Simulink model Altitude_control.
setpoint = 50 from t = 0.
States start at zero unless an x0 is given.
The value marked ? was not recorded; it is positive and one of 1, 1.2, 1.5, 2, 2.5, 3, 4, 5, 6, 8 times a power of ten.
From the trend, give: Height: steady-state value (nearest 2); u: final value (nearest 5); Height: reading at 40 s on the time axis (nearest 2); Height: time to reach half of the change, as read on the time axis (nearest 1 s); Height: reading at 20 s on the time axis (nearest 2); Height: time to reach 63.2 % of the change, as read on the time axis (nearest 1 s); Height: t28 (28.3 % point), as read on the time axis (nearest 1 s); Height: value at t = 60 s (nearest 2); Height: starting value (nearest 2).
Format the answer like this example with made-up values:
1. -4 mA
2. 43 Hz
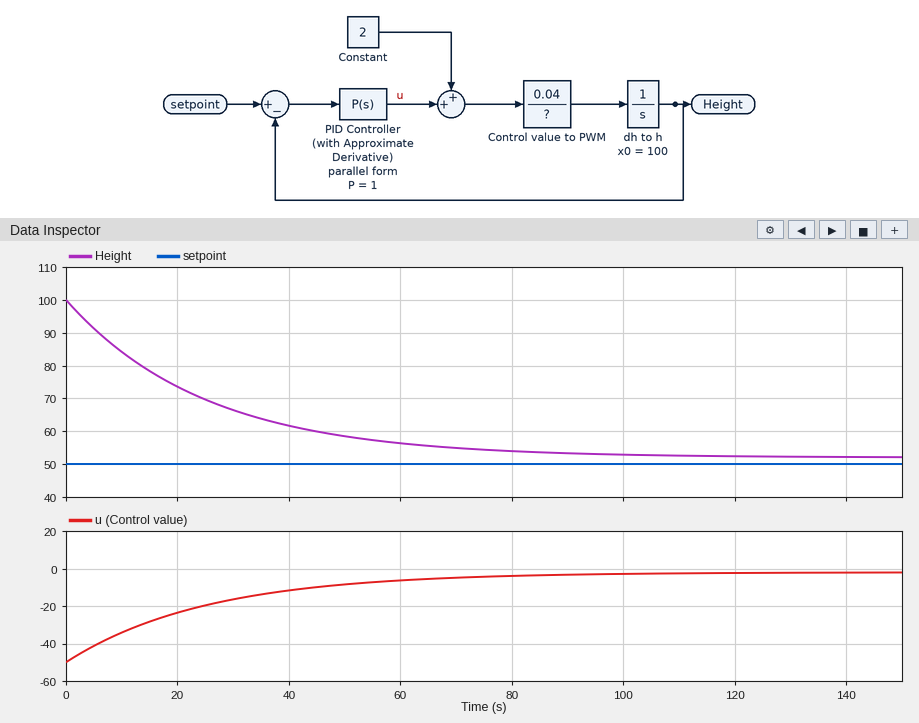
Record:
1. 52
2. 0
3. 62
4. 17 s
5. 74
6. 25 s
7. 8 s
8. 56
9. 100
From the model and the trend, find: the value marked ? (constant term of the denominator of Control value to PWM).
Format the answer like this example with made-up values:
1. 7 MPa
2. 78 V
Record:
1. 1
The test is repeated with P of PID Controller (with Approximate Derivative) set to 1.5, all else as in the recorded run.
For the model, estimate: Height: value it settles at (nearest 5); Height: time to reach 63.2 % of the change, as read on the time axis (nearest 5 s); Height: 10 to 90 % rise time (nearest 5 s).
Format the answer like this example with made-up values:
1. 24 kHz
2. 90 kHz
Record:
1. 50
2. 15 s
3. 35 s
